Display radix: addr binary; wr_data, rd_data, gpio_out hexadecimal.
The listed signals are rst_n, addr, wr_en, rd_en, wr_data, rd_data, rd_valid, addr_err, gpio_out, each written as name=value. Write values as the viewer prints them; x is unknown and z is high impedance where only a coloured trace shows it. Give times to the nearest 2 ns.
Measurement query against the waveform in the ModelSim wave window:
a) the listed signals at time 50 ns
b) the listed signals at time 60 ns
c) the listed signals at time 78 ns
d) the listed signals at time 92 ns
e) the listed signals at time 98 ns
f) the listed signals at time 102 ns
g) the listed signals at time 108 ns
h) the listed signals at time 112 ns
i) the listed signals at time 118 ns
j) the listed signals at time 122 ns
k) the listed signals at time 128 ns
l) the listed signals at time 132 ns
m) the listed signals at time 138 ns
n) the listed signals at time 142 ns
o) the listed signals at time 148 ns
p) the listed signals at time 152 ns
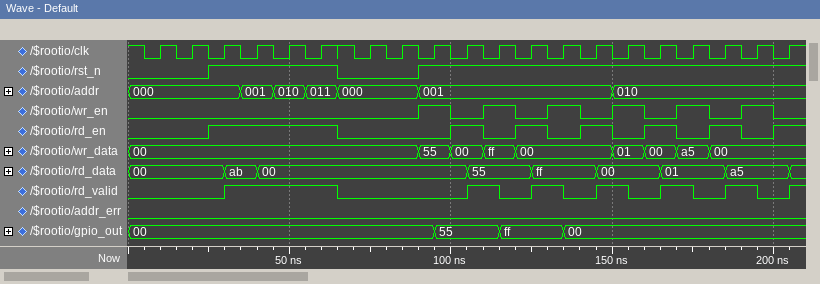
rst_n=1, addr=010, wr_en=0, rd_en=1, wr_data=00, rd_data=00, rd_valid=1, addr_err=0, gpio_out=00
rst_n=1, addr=011, wr_en=0, rd_en=1, wr_data=00, rd_data=00, rd_valid=1, addr_err=0, gpio_out=00
rst_n=0, addr=000, wr_en=0, rd_en=0, wr_data=00, rd_data=00, rd_valid=0, addr_err=0, gpio_out=00
rst_n=1, addr=001, wr_en=1, rd_en=0, wr_data=55, rd_data=00, rd_valid=0, addr_err=0, gpio_out=00
rst_n=1, addr=001, wr_en=1, rd_en=0, wr_data=55, rd_data=00, rd_valid=0, addr_err=0, gpio_out=55
rst_n=1, addr=001, wr_en=0, rd_en=1, wr_data=00, rd_data=00, rd_valid=0, addr_err=0, gpio_out=55
rst_n=1, addr=001, wr_en=0, rd_en=1, wr_data=00, rd_data=55, rd_valid=1, addr_err=0, gpio_out=55
rst_n=1, addr=001, wr_en=1, rd_en=0, wr_data=ff, rd_data=55, rd_valid=1, addr_err=0, gpio_out=55
rst_n=1, addr=001, wr_en=1, rd_en=0, wr_data=ff, rd_data=55, rd_valid=0, addr_err=0, gpio_out=ff
rst_n=1, addr=001, wr_en=0, rd_en=1, wr_data=00, rd_data=55, rd_valid=0, addr_err=0, gpio_out=ff
rst_n=1, addr=001, wr_en=0, rd_en=1, wr_data=00, rd_data=ff, rd_valid=1, addr_err=0, gpio_out=ff
rst_n=1, addr=001, wr_en=1, rd_en=0, wr_data=00, rd_data=ff, rd_valid=1, addr_err=0, gpio_out=ff
rst_n=1, addr=001, wr_en=1, rd_en=0, wr_data=00, rd_data=ff, rd_valid=0, addr_err=0, gpio_out=00
rst_n=1, addr=001, wr_en=0, rd_en=1, wr_data=00, rd_data=ff, rd_valid=0, addr_err=0, gpio_out=00
rst_n=1, addr=001, wr_en=0, rd_en=1, wr_data=00, rd_data=00, rd_valid=1, addr_err=0, gpio_out=00
rst_n=1, addr=010, wr_en=1, rd_en=0, wr_data=01, rd_data=00, rd_valid=1, addr_err=0, gpio_out=00
